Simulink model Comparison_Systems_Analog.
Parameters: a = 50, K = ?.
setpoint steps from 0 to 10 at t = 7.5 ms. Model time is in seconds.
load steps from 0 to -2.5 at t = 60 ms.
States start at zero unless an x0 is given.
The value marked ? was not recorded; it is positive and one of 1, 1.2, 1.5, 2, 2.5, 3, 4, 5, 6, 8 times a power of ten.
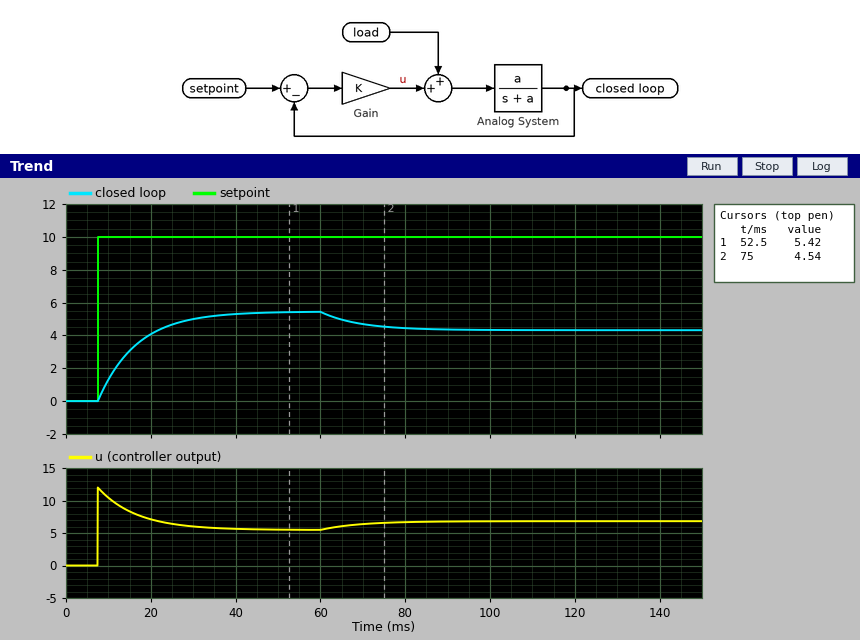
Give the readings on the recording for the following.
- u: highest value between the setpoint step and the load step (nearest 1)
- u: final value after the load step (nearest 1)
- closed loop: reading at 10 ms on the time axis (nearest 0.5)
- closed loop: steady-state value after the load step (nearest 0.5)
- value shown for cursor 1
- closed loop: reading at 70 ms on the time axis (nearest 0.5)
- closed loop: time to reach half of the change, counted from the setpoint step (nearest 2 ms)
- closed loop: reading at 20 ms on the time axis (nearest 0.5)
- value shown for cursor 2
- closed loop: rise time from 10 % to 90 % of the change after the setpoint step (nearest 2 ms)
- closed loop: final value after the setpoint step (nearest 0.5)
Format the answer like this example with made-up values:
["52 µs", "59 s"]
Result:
["12", "7", "1.5", "4.5", "5.42", "4.5", "6 ms", "4.0", "4.54", "20 ms", "5.5"]
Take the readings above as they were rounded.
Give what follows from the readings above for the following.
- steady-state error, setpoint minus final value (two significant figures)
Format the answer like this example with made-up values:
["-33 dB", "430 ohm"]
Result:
["4.5"]
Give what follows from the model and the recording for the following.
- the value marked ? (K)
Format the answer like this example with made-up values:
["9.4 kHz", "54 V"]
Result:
["1.2"]
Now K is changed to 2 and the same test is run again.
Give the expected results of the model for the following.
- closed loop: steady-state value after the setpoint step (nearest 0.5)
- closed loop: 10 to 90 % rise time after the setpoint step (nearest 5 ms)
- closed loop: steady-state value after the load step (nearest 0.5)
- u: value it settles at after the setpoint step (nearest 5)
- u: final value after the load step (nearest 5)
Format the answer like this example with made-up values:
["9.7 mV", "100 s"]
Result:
["6.5", "15 ms", "6.0", "5", "10"]
